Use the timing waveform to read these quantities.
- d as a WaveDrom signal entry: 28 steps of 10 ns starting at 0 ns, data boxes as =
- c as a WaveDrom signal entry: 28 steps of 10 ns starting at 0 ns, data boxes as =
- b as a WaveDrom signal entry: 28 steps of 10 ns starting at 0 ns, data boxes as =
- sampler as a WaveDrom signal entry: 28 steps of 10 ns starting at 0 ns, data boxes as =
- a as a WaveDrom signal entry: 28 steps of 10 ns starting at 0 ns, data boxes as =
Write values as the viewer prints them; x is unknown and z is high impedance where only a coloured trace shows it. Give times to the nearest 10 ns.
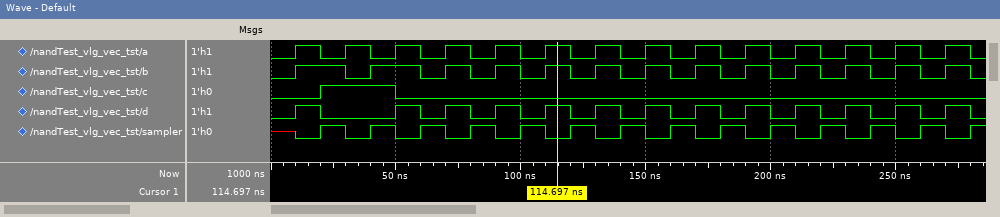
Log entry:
{name: 'd', wave: '010..10101010101010101010101'}
{name: 'c', wave: '0.1..0......................'}
{name: 'b', wave: '01.01.0101010101010101010101'}
{name: 'sampler', wave: 'x010101010101010101010101010'}
{name: 'a', wave: '0101010101010101010101010101'}
